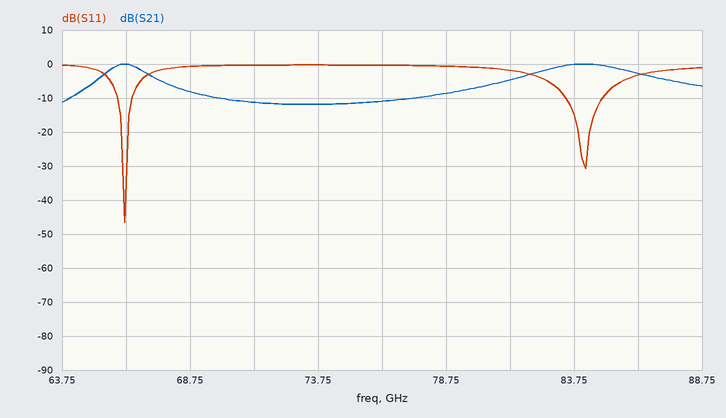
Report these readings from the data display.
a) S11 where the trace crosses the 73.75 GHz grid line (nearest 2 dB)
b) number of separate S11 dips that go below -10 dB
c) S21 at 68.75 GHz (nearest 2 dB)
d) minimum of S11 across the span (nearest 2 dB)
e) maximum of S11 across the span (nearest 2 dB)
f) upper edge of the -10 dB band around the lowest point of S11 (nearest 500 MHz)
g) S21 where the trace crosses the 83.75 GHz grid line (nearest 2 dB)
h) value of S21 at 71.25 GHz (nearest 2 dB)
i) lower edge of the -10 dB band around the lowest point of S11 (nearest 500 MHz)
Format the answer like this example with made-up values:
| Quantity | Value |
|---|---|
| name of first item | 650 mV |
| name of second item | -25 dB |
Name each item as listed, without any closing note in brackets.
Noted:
| Quantity | Value |
|---|---|
| S11 where the trace crosses the 73.75 GHz grid line | 0 dB |
| number of separate S11 dips that go below -10 dB | 2 |
| S21 at 68.75 GHz | -8 dB |
| minimum of S11 across the span | -46 dB |
| maximum of S11 across the span | 0 dB |
| upper edge of the -10 dB band around the lowest point of S11 | 66.5 GHz |
| S21 where the trace crosses the 83.75 GHz grid line | 0 dB |
| value of S21 at 71.25 GHz | -12 dB |
| lower edge of the -10 dB band around the lowest point of S11 | 66.0 GHz |
